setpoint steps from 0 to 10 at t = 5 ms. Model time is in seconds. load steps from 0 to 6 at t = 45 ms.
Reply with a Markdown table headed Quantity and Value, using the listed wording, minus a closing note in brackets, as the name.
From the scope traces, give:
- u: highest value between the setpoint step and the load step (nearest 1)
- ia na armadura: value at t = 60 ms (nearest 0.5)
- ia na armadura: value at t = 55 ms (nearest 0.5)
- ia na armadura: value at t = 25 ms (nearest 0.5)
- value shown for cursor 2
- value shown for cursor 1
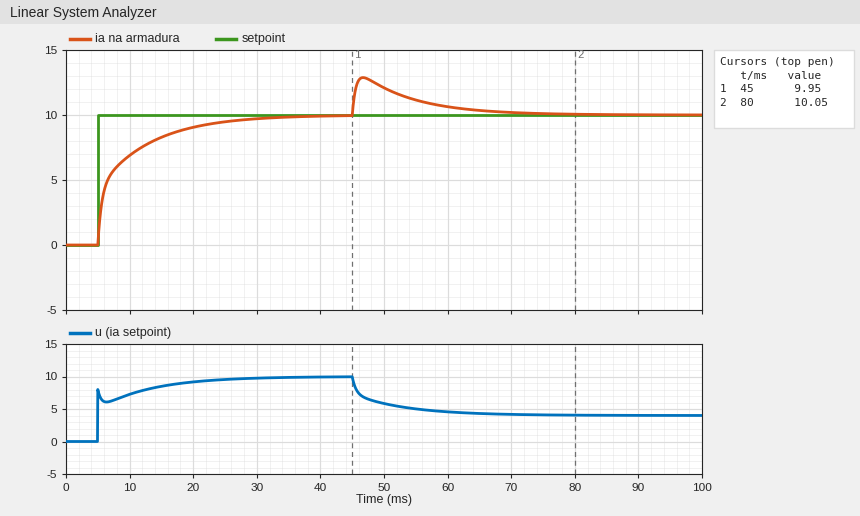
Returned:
| Quantity | Value |
|---|---|
| u: highest value between the setpoint step and the load step | 10 |
| ia na armadura: value at t = 60 ms | 10.5 |
| ia na armadura: value at t = 55 ms | 11.0 |
| ia na armadura: value at t = 25 ms | 9.5 |
| value shown for cursor 2 | 10.05 |
| value shown for cursor 1 | 9.95 |
